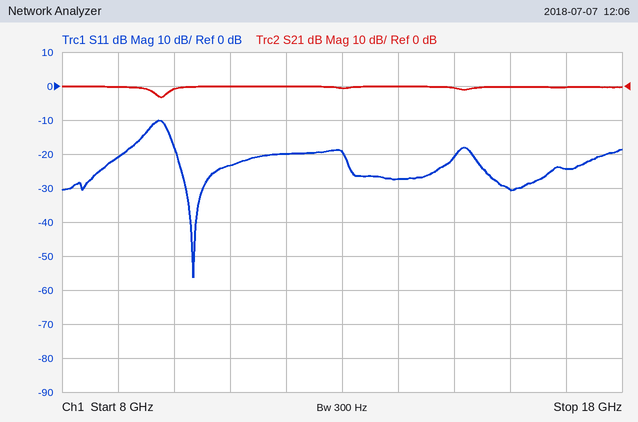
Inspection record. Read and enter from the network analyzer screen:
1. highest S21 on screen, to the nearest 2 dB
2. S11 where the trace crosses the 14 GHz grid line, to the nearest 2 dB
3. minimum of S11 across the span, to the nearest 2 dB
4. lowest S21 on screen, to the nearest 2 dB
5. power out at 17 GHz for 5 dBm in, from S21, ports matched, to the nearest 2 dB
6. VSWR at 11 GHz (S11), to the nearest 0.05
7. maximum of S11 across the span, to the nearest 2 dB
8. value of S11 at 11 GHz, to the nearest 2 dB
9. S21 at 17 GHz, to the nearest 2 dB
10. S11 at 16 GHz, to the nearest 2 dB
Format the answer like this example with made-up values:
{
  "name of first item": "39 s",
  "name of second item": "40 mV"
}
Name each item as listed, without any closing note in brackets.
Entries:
{
  "highest S21 on screen, to the nearest 2 dB": "0 dB",
  "S11 where the trace crosses the 14 GHz grid line, to the nearest 2 dB": "-28 dB",
  "minimum of S11 across the span, to the nearest 2 dB": "-56 dB",
  "lowest S21 on screen, to the nearest 2 dB": "-4 dB",
  "power out at 17 GHz for 5 dBm in, from S21, ports matched, to the nearest 2 dB": "4 dBm",
  "VSWR at 11 GHz (S11), to the nearest 0.05": "1.15",
  "maximum of S11 across the span, to the nearest 2 dB": "-10 dB",
  "value of S11 at 11 GHz, to the nearest 2 dB": "-24 dB",
  "S21 at 17 GHz, to the nearest 2 dB": "0 dB",
  "S11 at 16 GHz, to the nearest 2 dB": "-30 dB"
}
